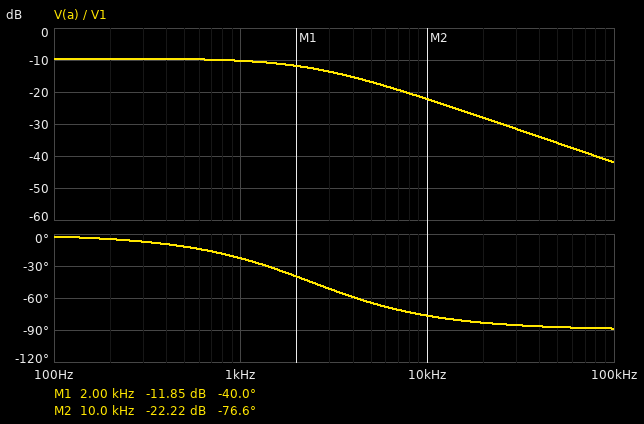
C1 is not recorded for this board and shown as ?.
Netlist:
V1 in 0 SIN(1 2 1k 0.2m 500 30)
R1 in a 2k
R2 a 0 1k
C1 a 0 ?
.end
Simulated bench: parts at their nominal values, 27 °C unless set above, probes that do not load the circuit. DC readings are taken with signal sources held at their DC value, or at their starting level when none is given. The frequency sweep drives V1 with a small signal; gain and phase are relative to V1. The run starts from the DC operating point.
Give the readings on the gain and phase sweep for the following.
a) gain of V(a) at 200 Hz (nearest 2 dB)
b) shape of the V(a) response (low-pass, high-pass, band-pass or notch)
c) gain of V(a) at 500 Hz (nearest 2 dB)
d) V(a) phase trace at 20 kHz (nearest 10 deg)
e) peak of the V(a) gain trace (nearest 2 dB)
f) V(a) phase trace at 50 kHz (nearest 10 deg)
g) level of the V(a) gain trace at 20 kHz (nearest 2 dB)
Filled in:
-10 dB
low-pass
-10 dB
-80 deg
-10 dB
-90 deg
-28 dB
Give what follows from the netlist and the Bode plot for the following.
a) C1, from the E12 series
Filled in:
100 nF
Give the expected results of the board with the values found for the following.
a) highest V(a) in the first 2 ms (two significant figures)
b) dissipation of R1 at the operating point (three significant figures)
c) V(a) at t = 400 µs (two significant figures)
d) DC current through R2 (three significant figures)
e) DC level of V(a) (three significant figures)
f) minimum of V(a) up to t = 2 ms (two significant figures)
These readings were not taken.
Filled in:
910 mV
889 µW
910 mV
667 µA
667 mV
-110 mV
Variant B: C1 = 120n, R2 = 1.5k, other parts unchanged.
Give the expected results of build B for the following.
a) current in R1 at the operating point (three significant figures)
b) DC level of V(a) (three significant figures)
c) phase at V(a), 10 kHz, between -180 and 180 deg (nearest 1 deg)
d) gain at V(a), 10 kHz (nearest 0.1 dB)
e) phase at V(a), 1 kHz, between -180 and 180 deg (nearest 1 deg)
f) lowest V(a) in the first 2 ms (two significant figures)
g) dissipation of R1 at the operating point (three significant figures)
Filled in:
571 µA
857 mV
-81 deg
-23.7 dB
-33 deg
-83 mV
653 µW
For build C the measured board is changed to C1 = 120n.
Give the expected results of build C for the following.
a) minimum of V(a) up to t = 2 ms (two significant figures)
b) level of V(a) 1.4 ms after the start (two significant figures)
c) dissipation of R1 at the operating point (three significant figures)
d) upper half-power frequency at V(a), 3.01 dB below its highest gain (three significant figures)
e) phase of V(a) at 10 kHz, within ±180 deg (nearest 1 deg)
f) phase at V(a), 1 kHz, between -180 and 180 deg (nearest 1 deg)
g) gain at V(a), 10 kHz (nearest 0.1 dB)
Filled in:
-92 mV
660 mV
889 µW
1.99 kHz
-79 deg
-27 deg
-23.7 dB
